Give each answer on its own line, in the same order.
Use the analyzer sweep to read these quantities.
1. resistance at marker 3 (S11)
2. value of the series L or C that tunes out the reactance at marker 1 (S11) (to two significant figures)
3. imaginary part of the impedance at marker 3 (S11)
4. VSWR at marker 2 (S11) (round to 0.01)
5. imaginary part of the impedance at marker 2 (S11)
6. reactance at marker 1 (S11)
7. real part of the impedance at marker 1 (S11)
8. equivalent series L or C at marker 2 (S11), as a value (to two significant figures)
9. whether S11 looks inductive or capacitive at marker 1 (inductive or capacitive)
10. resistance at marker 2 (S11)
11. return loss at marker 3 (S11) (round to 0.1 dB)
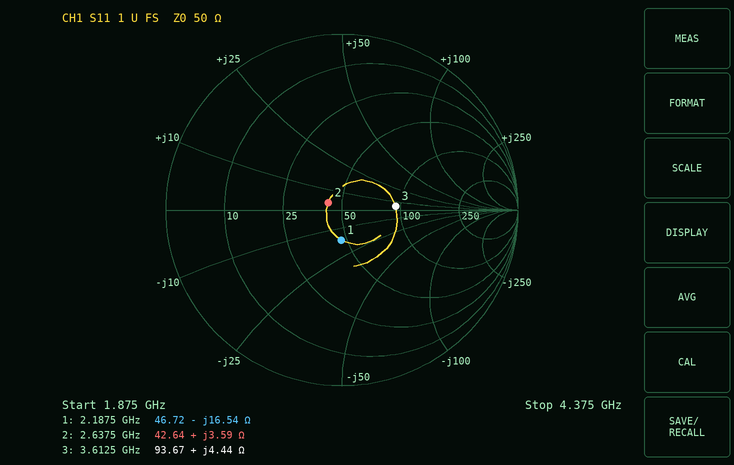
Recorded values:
93.67 Ω
1.2 nH
+4.44 Ω
1.19
+3.59 Ω
-16.54 Ω
46.72 Ω
220 pH
capacitive
42.64 Ω
10.3 dB
